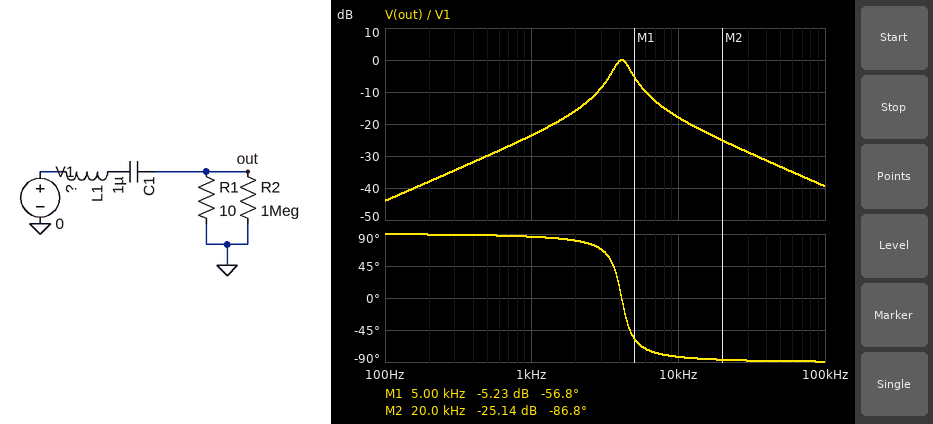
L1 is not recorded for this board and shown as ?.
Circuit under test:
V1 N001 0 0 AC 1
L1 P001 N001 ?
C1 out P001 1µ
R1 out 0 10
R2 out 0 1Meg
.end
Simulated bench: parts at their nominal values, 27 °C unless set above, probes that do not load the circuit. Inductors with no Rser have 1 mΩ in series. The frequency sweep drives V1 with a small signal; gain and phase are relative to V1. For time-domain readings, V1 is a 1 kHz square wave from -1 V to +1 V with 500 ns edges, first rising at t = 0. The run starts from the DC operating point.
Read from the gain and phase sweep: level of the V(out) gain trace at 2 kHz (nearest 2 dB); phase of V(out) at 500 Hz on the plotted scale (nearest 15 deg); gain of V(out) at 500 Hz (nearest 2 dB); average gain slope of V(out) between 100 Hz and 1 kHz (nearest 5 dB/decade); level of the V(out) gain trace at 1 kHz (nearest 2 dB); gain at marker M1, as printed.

-16 dB
90 deg
-30 dB
20 dB/decade
-24 dB
-5.23 dB
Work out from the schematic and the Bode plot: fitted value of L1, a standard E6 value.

1.5 mH
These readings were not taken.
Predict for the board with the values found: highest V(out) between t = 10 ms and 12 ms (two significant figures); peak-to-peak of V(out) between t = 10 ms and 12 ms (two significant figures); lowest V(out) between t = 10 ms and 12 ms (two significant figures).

360 mV
720 mV
-360 mV
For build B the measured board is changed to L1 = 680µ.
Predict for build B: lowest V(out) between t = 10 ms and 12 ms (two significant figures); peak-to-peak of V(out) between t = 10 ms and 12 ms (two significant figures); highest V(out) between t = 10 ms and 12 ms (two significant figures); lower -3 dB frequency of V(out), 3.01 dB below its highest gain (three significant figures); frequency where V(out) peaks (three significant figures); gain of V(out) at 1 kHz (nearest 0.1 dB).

-570 mV
1.1 V
570 mV
5.04 kHz
6.10 kHz
-23.8 dB
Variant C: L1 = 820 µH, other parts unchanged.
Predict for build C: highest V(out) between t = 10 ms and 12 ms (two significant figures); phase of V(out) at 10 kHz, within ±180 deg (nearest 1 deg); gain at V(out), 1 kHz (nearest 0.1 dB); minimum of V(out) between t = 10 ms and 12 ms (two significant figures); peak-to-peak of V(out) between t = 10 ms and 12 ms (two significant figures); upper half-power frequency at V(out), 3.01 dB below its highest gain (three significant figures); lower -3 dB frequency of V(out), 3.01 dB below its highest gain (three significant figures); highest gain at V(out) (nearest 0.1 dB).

550 mV
-74 deg
-23.8 dB
-550 mV
1.1 V
6.61 kHz
4.67 kHz
0 dB
